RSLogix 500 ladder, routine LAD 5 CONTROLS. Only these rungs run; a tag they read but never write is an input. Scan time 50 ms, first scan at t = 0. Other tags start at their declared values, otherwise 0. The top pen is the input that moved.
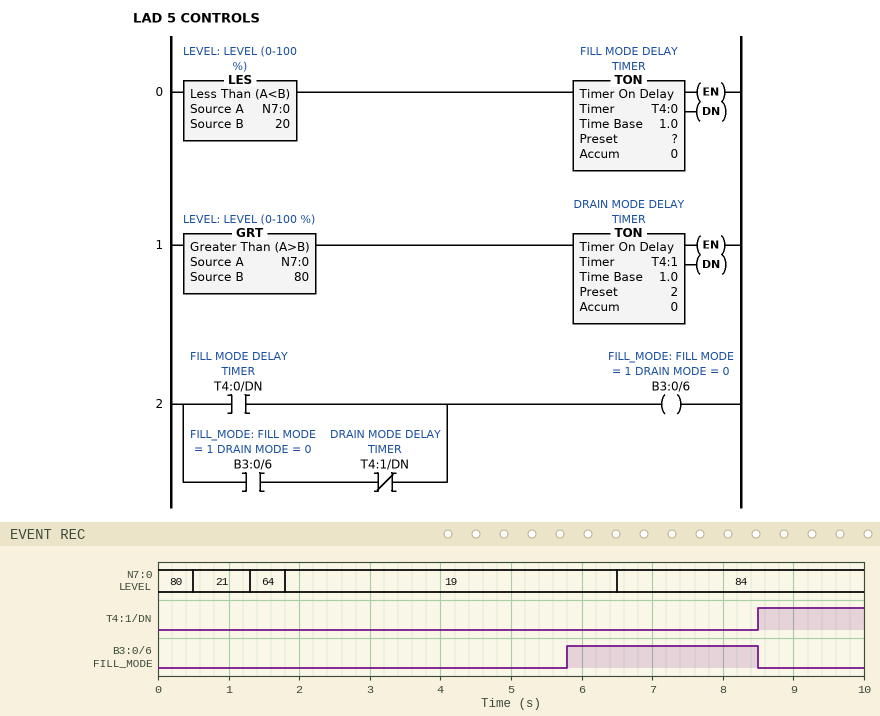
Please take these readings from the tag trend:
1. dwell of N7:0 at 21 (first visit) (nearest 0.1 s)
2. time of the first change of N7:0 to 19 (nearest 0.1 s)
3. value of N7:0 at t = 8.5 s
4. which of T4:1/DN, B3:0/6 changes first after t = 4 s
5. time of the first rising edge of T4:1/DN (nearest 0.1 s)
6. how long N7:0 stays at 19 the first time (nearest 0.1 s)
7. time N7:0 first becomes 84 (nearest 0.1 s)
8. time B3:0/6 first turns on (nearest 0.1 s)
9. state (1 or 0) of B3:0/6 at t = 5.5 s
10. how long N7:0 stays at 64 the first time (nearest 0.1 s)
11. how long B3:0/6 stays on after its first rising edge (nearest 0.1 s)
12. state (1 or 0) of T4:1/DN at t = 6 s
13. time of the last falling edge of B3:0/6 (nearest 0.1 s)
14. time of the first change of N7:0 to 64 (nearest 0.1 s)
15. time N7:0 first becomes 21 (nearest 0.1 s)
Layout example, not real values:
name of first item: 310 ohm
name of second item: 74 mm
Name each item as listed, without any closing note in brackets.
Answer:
dwell of N7:0 at 21 (first visit): 0.8 s
time of the first change of N7:0 to 19: 1.8 s
value of N7:0 at t = 8.5 s: 84
which of T4:1/DN, B3:0/6 changes first after t = 4 s: B3:0/6
time of the first rising edge of T4:1/DN: 8.5 s
how long N7:0 stays at 19 the first time: 4.7 s
time N7:0 first becomes 84: 6.5 s
time B3:0/6 first turns on: 5.8 s
state (1 or 0) of B3:0/6 at t = 5.5 s: 0
how long N7:0 stays at 64 the first time: 0.5 s
how long B3:0/6 stays on after its first rising edge: 2.7 s
state (1 or 0) of T4:1/DN at t = 6 s: 0
time of the last falling edge of B3:0/6: 8.5 s
time of the first change of N7:0 to 64: 1.3 s
time N7:0 first becomes 21: 0.5 s
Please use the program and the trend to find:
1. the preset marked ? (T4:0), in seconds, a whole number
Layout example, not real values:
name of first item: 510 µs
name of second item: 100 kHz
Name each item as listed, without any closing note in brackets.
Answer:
the preset marked ? (T4:0), in seconds, a whole number: 4 s
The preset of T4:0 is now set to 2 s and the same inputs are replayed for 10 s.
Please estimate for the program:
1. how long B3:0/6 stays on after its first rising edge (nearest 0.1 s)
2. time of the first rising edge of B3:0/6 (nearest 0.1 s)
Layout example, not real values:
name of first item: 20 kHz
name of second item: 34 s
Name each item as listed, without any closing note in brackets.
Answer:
how long B3:0/6 stays on after its first rising edge: 4.7 s
time of the first rising edge of B3:0/6: 3.8 s
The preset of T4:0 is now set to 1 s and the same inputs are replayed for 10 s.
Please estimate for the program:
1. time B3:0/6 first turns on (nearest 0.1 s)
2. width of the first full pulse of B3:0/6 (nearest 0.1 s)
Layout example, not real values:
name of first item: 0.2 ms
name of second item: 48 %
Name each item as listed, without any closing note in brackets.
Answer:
time B3:0/6 first turns on: 2.8 s
width of the first full pulse of B3:0/6: 5.7 s
